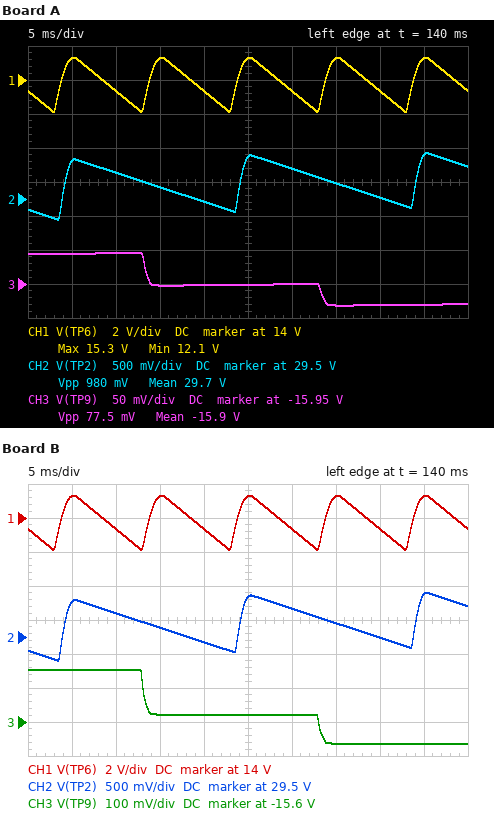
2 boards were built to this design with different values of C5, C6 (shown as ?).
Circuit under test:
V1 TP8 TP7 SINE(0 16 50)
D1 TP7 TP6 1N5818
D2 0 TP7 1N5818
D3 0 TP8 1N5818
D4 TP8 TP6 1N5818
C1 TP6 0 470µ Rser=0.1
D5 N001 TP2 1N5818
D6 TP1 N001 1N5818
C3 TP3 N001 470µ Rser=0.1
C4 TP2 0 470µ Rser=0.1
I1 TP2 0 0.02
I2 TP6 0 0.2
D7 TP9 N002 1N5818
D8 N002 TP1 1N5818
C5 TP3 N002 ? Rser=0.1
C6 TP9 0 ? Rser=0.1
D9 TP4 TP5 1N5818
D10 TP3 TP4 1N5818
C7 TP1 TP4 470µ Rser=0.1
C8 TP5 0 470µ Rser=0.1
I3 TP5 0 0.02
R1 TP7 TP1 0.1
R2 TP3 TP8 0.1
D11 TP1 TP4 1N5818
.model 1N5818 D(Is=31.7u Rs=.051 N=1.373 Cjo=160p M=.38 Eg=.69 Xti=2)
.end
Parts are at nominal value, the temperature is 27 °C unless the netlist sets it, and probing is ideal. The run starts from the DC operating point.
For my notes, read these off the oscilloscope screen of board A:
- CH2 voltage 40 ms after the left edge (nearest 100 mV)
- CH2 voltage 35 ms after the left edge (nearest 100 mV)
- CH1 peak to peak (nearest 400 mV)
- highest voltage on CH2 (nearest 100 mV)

29.5 V
29.7 V
3.2 V
30.2 V
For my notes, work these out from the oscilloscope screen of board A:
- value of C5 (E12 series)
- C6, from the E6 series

270 µF
220 µF
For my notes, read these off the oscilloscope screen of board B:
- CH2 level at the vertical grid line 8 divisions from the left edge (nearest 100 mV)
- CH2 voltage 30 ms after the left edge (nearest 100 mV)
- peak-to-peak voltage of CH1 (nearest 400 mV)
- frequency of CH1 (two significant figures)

29.5 V
29.9 V
3.2 V
100 Hz
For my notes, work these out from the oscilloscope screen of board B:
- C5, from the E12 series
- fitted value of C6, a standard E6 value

1.5 mF
1.5 mF
